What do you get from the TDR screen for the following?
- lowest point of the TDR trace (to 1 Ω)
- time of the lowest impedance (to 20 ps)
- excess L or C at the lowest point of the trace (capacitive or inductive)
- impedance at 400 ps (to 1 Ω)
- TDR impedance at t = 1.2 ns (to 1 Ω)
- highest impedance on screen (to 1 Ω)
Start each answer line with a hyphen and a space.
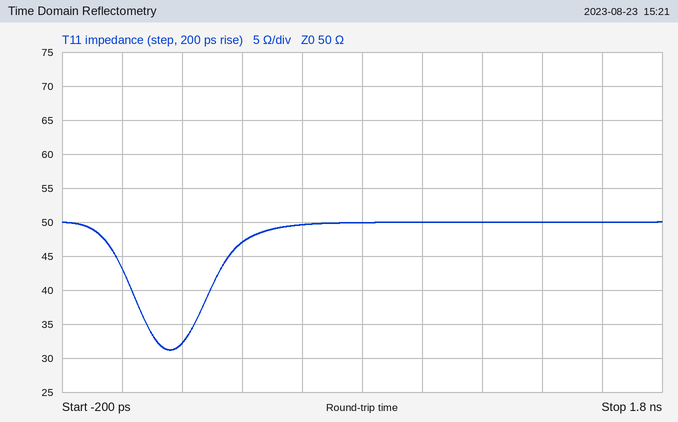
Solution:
- 31 Ω
- 160 ps
- capacitive
- 47 Ω
- 50 Ω
- 50 Ω
